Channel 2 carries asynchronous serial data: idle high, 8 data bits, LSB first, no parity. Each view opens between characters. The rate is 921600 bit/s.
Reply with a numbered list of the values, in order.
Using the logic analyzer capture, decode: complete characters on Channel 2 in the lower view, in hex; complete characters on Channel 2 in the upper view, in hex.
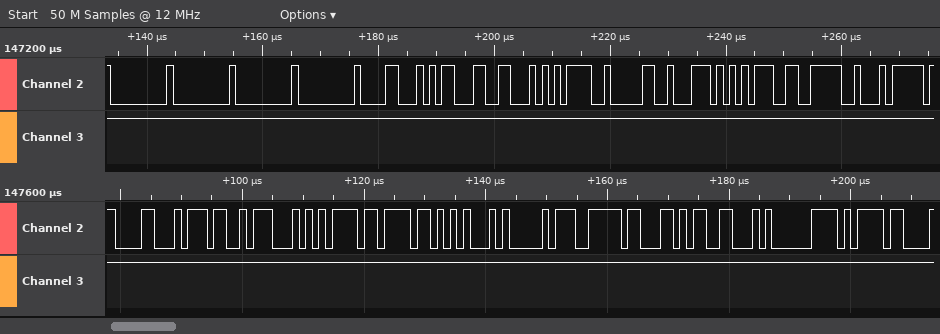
1. 18, 37, 47, BD, 6F, 45, D0, BE, AC, 46, E0, BD
2. 00, 00, 00, 00, 18, 8D, 46, 3D, 30, 5C, 9D, 3E, F4
